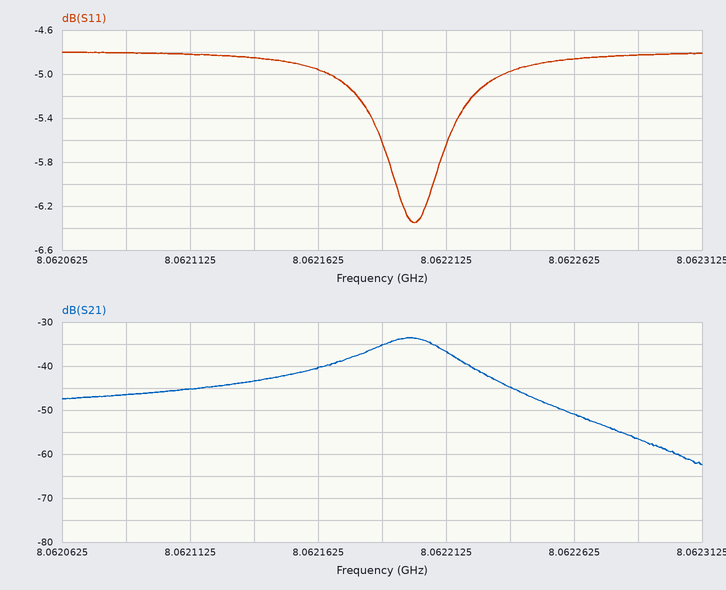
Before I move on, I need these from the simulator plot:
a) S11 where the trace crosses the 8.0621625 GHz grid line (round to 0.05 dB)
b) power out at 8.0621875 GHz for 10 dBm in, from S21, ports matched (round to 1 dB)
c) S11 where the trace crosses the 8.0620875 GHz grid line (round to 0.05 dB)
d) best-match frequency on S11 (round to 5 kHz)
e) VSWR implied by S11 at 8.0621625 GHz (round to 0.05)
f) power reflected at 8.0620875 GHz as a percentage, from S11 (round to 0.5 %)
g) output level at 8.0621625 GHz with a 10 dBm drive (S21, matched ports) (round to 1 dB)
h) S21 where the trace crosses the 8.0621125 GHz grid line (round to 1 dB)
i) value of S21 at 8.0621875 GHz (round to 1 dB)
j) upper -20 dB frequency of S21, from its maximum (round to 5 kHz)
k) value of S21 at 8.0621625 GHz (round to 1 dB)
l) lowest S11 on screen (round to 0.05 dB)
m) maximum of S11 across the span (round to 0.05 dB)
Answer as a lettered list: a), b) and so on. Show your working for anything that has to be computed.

a) -4.95 dB
b) 10 dBm + (-35 dB) = -25 dBm
c) -4.80 dB
d) 8.062200 GHz
e) |Γ| = 10^(-4.95/20) = 0.5656; VSWR = (1 + 0.5656)/(1 − 0.5656) ≈ 3.60
f) 10^(-4.8/10) ≈ 33.1 %, so 33.0 % to the nearest 0.5 %
g) 10 dBm + (-40 dB) = -30 dBm
h) -45 dB
i) -35 dB
j) 8.062275 GHz
k) -40 dB
l) -6.35 dB
m) -4.80 dB
